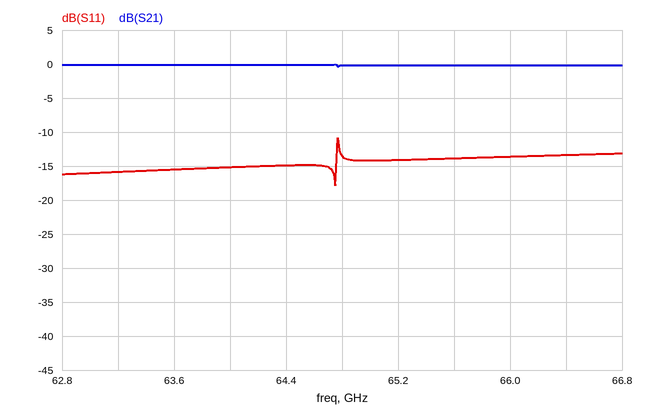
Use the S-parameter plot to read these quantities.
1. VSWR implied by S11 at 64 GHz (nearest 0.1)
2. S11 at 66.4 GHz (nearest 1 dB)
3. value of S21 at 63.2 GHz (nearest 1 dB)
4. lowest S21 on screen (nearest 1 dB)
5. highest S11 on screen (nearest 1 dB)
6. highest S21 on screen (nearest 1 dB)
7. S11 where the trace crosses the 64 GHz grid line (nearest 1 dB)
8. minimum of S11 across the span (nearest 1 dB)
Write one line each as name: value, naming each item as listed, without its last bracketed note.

VSWR implied by S11 at 64 GHz: 1.4
S11 at 66.4 GHz: -13 dB
value of S21 at 63.2 GHz: 0 dB
lowest S21 on screen: 0 dB
highest S11 on screen: -11 dB
highest S21 on screen: 0 dB
S11 where the trace crosses the 64 GHz grid line: -15 dB
minimum of S11 across the span: -18 dB
